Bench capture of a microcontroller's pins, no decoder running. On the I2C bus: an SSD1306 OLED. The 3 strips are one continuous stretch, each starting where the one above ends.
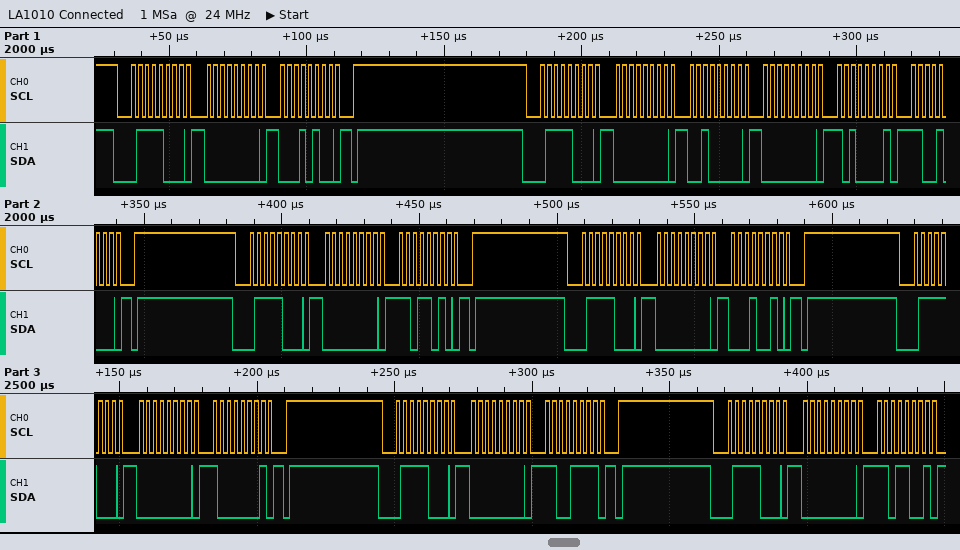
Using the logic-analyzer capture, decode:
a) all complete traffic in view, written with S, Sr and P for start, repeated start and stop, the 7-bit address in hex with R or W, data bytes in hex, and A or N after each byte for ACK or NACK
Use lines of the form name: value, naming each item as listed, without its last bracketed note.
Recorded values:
all complete traffic in view, written with S, Sr and P for start, repeated start and stop, the 7-bit address in hex with R or W, data bytes in hex, and A or N after each byte for ACK or NACK: S 3CW A 00 A 14 A P S 3CW A 00 A 20 A 00 A A1 A C8 A P S 3CW A 00 A DA A P S 3CW A 00 A 12 A P S 3CW A 00 A 81 A P S 3CW A 00 A CF A P S 3CW A 00 A D9 A
